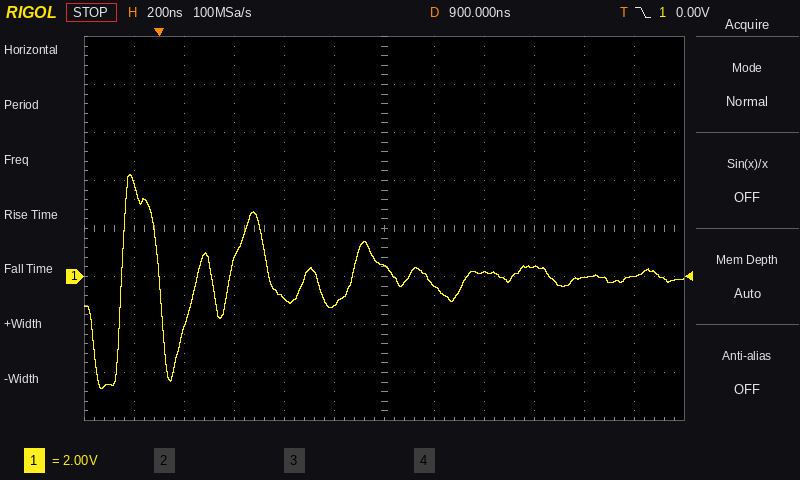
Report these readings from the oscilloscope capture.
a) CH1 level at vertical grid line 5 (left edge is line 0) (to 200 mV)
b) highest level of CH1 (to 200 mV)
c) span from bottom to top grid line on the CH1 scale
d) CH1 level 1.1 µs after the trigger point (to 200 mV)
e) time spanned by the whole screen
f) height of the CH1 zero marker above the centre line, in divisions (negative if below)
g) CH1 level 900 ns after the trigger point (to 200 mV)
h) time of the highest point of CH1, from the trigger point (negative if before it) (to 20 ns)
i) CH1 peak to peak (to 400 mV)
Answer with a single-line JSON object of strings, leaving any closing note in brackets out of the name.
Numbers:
{"CH1 level at vertical grid line 5 (left edge is line 0)": "-1.2 V", "highest level of CH1": "4.2 V", "span from bottom to top grid line on the CH1 scale": "16 V", "CH1 level 1.1 µs after the trigger point": "-400 mV", "time spanned by the whole screen": "2.4 µs", "height of the CH1 zero marker above the centre line, in divisions": "-1.0 div", "CH1 level 900 ns after the trigger point": "400 mV", "time of the highest point of CH1, from the trigger point (negative if before it)": "-120 ns", "CH1 peak to peak": "8.8 V"}
